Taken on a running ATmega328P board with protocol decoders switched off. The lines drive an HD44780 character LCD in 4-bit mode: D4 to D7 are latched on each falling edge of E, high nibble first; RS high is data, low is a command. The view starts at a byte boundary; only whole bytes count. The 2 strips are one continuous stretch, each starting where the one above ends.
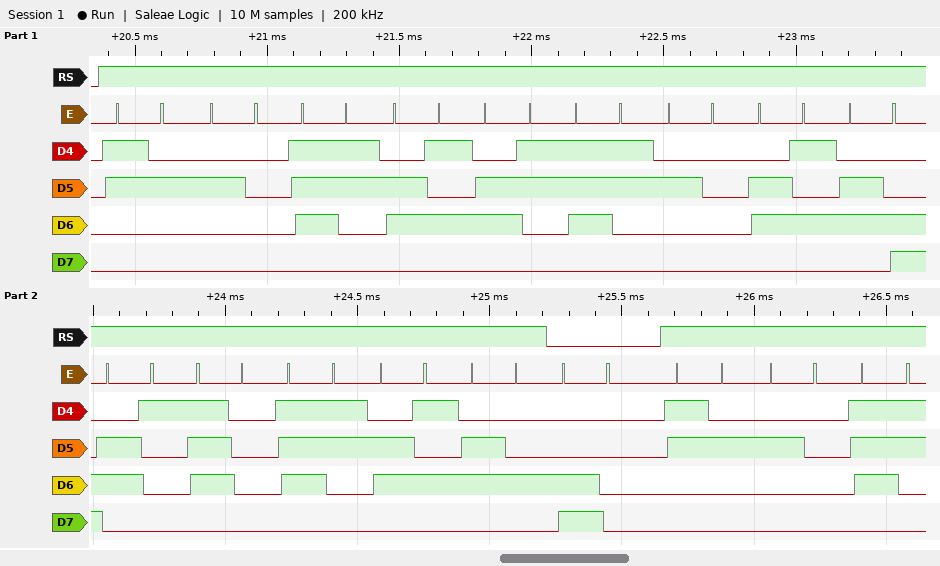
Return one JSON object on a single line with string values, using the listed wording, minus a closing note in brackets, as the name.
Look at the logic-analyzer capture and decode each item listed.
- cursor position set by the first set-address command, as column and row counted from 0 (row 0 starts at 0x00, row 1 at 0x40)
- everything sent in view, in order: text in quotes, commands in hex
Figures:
{"cursor position set by the first set-address command, as column and row counted from 0": "column 0, row 1", "everything sent in view, in order: text in quotes, commands in hex": "\"2 secs elapsed\" 0xC0 \"2 s\""}
